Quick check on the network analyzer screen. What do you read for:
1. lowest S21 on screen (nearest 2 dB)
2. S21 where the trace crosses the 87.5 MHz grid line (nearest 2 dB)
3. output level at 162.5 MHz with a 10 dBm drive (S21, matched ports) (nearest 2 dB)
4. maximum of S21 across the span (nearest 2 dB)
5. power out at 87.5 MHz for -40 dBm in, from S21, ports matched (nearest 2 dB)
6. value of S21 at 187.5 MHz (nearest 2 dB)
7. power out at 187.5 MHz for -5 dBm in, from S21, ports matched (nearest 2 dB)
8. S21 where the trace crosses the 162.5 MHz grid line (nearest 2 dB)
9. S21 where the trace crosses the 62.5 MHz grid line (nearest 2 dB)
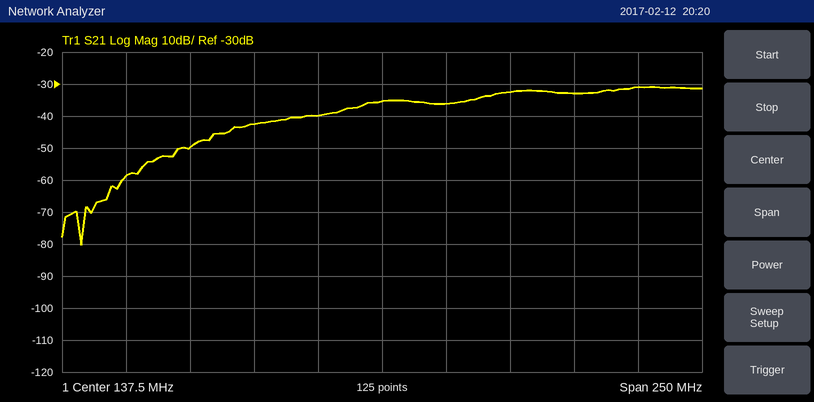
-80 dB
-42 dB
-26 dBm
-30 dB
-82 dBm
-32 dB
-38 dBm
-36 dB
-50 dB
